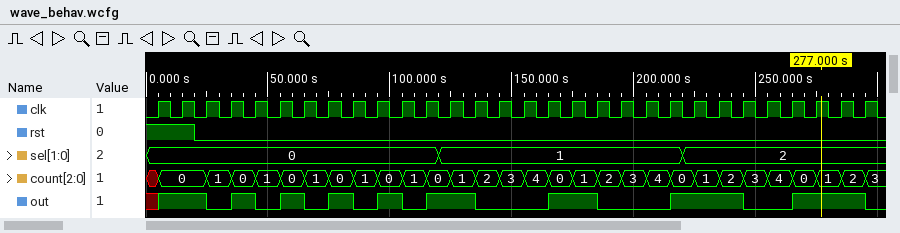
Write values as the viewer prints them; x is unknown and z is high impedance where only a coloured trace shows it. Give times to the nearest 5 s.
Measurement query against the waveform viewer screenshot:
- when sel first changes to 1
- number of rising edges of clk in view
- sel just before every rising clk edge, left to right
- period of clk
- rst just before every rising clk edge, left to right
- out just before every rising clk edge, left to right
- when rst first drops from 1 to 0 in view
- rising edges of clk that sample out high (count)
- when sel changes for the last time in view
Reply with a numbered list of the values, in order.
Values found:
1. 120 s
2. 30
3. 0, 0, 0, 0, 0, 0, 0, 0, 0, 0, 0, 0, 1, 1, 1, 1, 1, 1, 1, 1, 1, 1, 2, 2, 2, 2, 2, 2, 2, 2
4. 10 s
5. 1 1 0 0 0 0 0 0 0 0 0 0 0 0 0 0 0 0 0 0 0 0 0 0 0 0 0 0 0 0
6. x 1 1 0 1 0 1 0 1 0 1 0 1 1 0 0 0 1 1 0 0 0 1 1 1 0 0 1 1 1
7. 20 s
8. 16
9. 220 s
